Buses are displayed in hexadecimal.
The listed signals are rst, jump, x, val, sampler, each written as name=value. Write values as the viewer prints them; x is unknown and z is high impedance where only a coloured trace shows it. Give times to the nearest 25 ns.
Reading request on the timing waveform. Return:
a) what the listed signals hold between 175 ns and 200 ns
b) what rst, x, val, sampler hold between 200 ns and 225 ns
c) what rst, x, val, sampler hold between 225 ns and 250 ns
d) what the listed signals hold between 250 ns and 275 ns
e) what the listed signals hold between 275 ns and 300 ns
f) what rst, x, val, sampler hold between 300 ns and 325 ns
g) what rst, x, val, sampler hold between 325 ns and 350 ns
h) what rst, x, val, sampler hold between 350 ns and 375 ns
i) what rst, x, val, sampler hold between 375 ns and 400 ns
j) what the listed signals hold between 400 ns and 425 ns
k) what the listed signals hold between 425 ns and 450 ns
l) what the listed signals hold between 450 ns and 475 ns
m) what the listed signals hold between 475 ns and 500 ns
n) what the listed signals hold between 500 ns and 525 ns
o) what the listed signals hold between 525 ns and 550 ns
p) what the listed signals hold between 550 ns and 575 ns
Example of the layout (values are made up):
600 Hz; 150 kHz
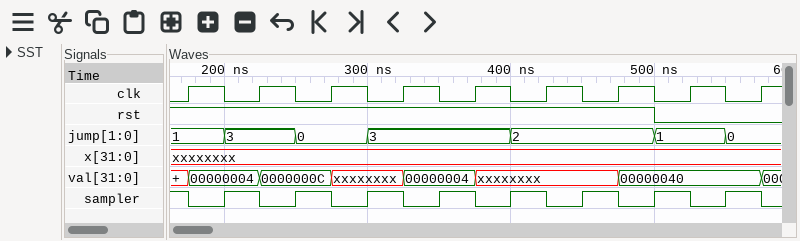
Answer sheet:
rst=1, jump=1, x=xxxxxxxx, val=00000004, sampler=0; rst=1, x=xxxxxxxx, val=00000004, sampler=1; rst=1, x=xxxxxxxx, val=0000000C, sampler=0; rst=1, jump=0, x=xxxxxxxx, val=0000000C, sampler=1; rst=1, jump=0, x=xxxxxxxx, val=xxxxxxxx, sampler=0; rst=1, x=xxxxxxxx, val=xxxxxxxx, sampler=1; rst=1, x=xxxxxxxx, val=00000004, sampler=0; rst=1, x=xxxxxxxx, val=00000004, sampler=1; rst=1, x=xxxxxxxx, val=xxxxxxxx, sampler=0; rst=1, jump=2, x=xxxxxxxx, val=xxxxxxxx, sampler=1; rst=1, jump=2, x=xxxxxxxx, val=xxxxxxxx, sampler=0; rst=1, jump=2, x=xxxxxxxx, val=xxxxxxxx, sampler=1; rst=1, jump=2, x=xxxxxxxx, val=00000040, sampler=0; rst=0, jump=1, x=xxxxxxxx, val=00000040, sampler=1; rst=0, jump=1, x=xxxxxxxx, val=00000040, sampler=0; rst=0, jump=0, x=xxxxxxxx, val=00000040, sampler=1
